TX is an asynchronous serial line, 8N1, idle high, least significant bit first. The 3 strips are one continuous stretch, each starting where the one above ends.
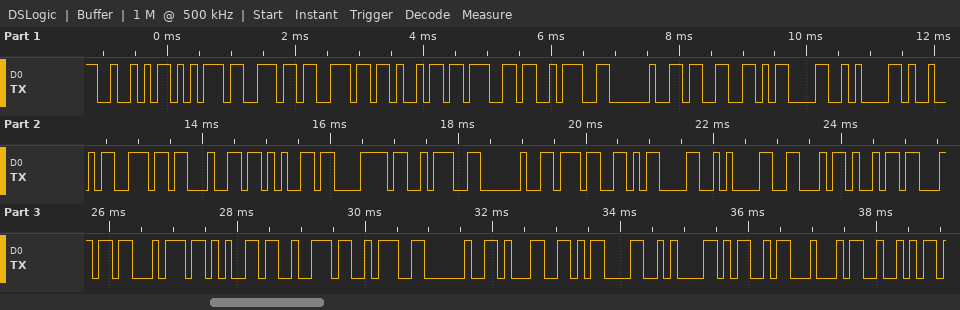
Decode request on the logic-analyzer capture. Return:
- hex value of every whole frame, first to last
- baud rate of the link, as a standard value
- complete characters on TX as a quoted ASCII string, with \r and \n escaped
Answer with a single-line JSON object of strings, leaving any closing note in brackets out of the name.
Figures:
{"hex value of every whole frame, first to last": "0x52 0x75 0x6E 0x6E 0x69 0x67 0x3A 0x20 0x33 0x0D 0x0A 0x49 0x6E 0x64 0x65 0x78 0x3A 0x20 0x37 0x0D 0x0A 0x46 0x69 0x6C 0x74 0x65 0x72 0x3A 0x20 0x31 0x0D 0x0A 0x4D 0x44 0x52", "baud rate of the link, as a standard value": "9600 baud", "complete characters on TX as a quoted ASCII string, with \\r and \\n escaped": "\"Runnig: 3\\r\\nIndex: 7\\r\\nFilter: 1\\r\\nMDR\""}
